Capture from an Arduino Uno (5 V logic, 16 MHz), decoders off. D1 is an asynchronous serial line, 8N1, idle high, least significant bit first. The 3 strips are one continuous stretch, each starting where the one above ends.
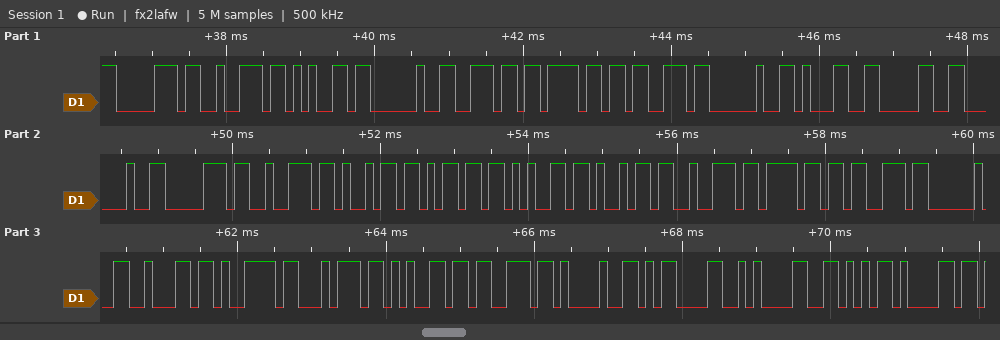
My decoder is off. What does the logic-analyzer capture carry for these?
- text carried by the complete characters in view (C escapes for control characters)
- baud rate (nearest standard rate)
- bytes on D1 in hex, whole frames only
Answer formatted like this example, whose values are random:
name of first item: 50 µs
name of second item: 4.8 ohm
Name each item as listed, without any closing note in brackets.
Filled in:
text carried by the complete characters in view: "pre nos 10 primeiros bytes!\r\nVa"
baud rate: 9600 baud
bytes on D1 in hex, whole frames only: 70 72 65 20 6E 6F 73 20 31 30 20 70 72 69 6D 65 69 72 6F 73 20 62 79 74 65 73 21 0D 0A 56 61
